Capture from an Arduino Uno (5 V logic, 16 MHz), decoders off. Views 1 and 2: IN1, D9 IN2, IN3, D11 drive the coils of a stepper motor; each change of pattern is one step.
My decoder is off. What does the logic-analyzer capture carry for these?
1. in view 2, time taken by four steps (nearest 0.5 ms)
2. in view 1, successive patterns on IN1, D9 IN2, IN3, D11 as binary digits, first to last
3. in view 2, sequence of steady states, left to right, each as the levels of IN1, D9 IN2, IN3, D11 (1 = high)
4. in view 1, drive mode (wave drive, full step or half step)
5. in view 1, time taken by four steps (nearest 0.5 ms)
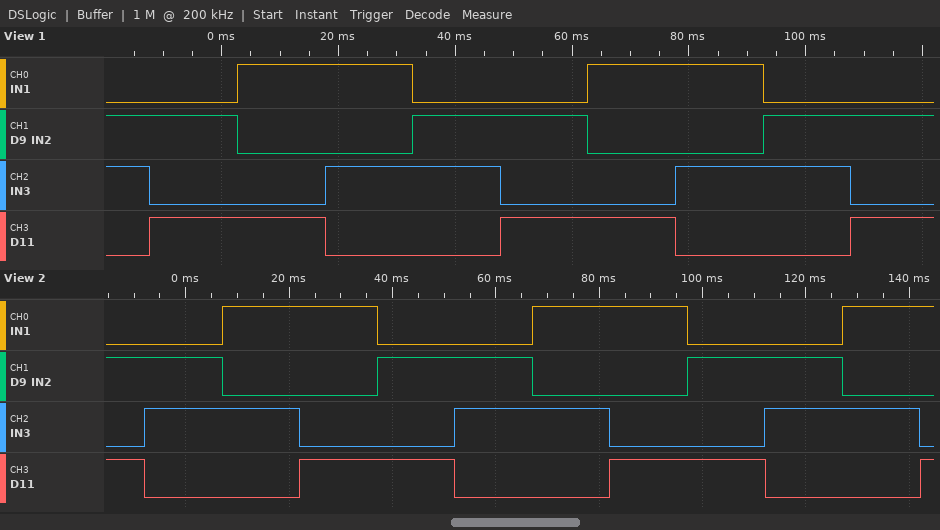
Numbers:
60.0 ms
0110 0101 1001 1010 0110 0101 1001 1010 0110 0101
0101 0110 1010 1001 0101 0110 1010 1001 0101 0110 1010 1001
full step
60.0 ms
